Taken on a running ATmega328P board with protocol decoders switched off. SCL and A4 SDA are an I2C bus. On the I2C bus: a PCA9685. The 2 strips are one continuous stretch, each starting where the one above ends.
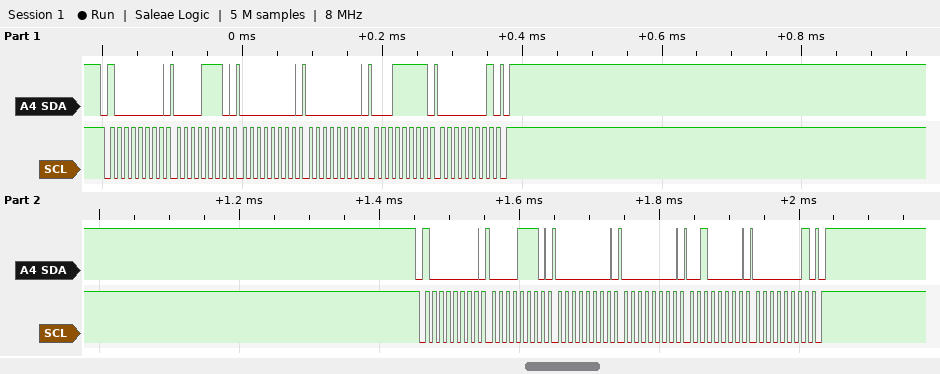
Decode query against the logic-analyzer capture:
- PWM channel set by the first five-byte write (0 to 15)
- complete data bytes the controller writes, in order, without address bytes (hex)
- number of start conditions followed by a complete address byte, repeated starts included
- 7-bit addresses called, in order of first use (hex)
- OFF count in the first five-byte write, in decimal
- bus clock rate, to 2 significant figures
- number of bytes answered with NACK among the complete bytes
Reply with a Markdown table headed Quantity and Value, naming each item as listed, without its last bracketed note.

| Quantity | Value |
|---|---|
| PWM channel set by the first five-byte write | 2 |
| complete data bytes the controller writes, in order, without address bytes | 0E 00 00 1F 01 0E 00 00 20 01 |
| number of start conditions followed by a complete address byte, repeated starts included | 2 |
| 7-bit addresses called, in order of first use | 0x40 |
| OFF count in the first five-byte write, in decimal | 287 |
| bus clock rate, to 2 significant figures | 100 kHz |
| number of bytes answered with NACK among the complete bytes | 0 |
